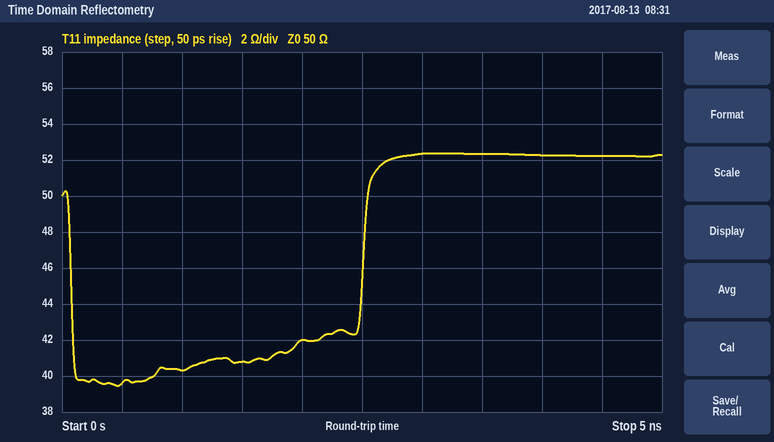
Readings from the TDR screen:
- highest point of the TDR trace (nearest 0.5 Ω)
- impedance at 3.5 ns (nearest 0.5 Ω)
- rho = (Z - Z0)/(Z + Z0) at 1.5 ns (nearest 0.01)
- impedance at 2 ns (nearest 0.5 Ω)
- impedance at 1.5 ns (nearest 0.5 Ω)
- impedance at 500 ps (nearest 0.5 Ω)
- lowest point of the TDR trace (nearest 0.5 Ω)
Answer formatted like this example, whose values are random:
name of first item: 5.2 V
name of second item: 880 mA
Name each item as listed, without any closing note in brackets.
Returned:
highest point of the TDR trace: 52.5 Ω
impedance at 3.5 ns: 52.5 Ω
rho = (Z - Z0)/(Z + Z0) at 1.5 ns: -0.10
impedance at 2 ns: 42.0 Ω
impedance at 1.5 ns: 41.0 Ω
impedance at 500 ps: 39.5 Ω
lowest point of the TDR trace: 39.5 Ω
